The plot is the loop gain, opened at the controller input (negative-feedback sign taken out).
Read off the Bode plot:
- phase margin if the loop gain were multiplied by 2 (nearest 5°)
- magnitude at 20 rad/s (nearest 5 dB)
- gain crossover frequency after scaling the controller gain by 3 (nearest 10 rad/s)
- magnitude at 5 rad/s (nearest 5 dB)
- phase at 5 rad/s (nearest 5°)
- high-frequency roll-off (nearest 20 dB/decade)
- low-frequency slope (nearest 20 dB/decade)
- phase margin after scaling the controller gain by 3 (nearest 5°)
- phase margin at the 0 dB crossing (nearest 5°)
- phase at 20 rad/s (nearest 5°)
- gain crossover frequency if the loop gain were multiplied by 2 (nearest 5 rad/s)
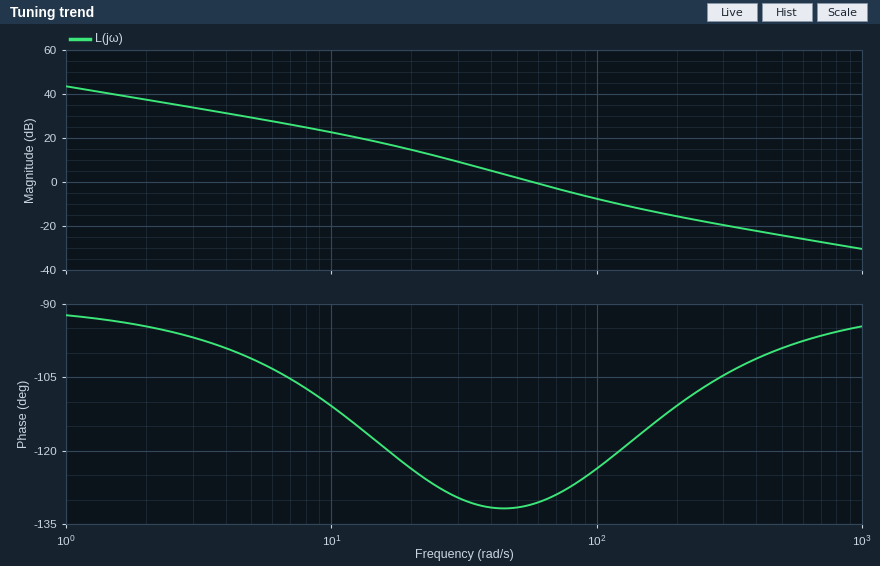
55°
15 dB
120 rad/s
30 dB
-100°
-20 dB/decade
-20 dB/decade
60°
50°
-125°
90 rad/s
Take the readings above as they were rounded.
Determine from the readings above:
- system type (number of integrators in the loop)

1
